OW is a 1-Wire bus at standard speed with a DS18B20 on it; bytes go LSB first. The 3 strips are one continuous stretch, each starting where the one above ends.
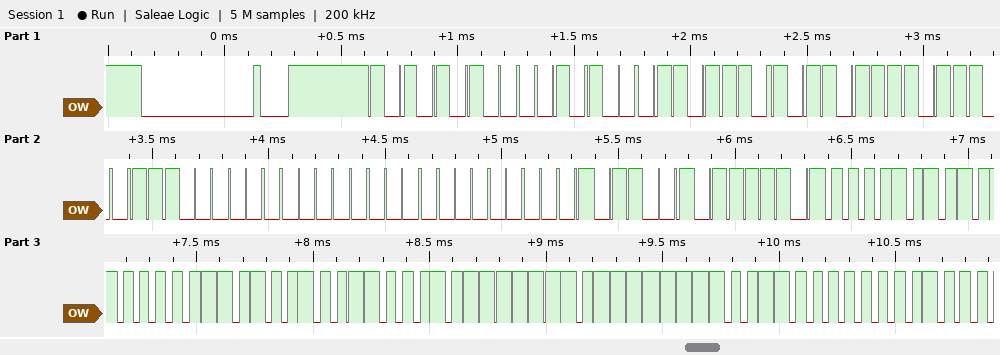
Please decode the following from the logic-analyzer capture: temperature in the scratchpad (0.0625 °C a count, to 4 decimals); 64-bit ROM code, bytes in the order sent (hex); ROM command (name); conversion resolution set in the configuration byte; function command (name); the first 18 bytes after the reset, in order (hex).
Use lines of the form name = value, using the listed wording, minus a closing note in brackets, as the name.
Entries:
temperature in the scratchpad = 85.0000 °C
64-bit ROM code, bytes in the order sent = 28 76 ED 9D 03 00 00 9A
ROM command = Match ROM
conversion resolution set in the configuration byte = 12 bits
function command = Read Scratchpad
the first 18 bytes after the reset, in order = 55 28 76 ED 9D 03 00 00 9A BE 50 05 4B 46 7F FF 0C 10
